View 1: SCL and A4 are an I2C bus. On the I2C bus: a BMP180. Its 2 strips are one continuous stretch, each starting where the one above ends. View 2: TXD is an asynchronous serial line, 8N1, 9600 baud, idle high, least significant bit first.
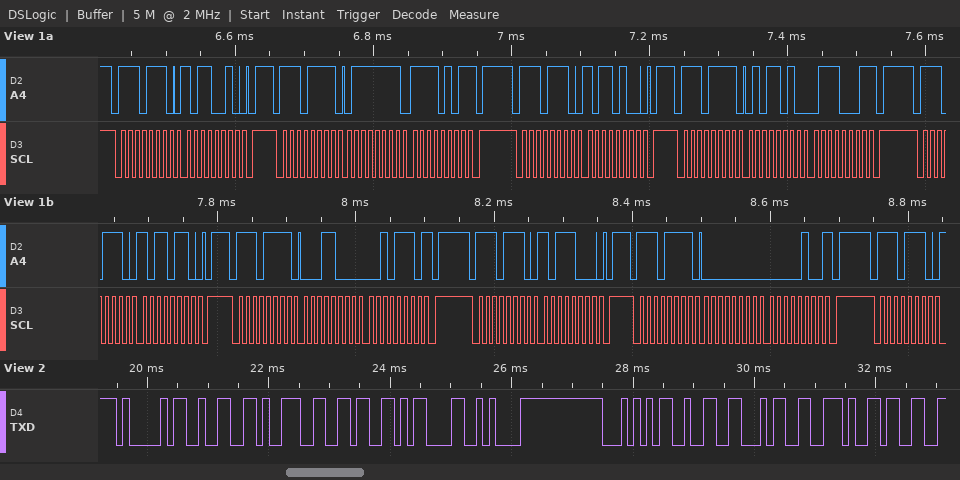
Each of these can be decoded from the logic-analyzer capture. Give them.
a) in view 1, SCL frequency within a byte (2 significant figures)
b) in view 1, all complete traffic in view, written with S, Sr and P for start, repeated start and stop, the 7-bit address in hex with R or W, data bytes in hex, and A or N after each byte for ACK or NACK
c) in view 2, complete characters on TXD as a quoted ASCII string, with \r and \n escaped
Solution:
100 kHz
S 77W A B2 A P S 77R A 7F A F5 N P S 77W A B4 A P S 77R A 5A A 71 N P S 77W A B6 A P S 77R A 18 A 2E N P S 77W A B8 A P S 77R A 00 A 04 N P S 77W A
"A296\r\nT24.3"
